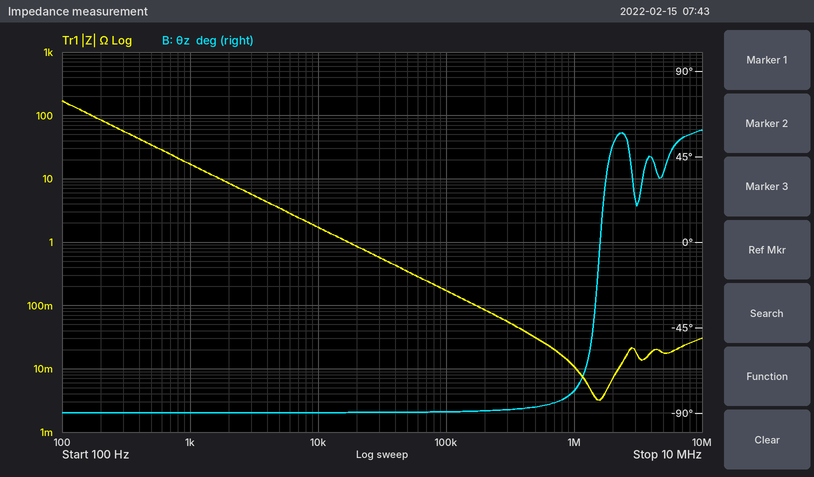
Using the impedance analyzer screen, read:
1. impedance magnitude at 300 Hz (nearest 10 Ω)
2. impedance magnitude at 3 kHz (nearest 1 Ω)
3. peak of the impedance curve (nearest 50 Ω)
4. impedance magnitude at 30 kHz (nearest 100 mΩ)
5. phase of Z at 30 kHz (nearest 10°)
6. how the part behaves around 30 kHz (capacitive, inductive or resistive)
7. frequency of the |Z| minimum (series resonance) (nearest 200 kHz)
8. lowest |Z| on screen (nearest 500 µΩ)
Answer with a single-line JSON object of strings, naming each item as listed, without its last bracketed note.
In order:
{"impedance magnitude at 300 Hz": "60 Ω", "impedance magnitude at 3 kHz": "6 Ω", "peak of the impedance curve": "150 Ω", "impedance magnitude at 30 kHz": "600 mΩ", "phase of Z at 30 kHz": "-90°", "how the part behaves around 30 kHz": "capacitive", "frequency of the |Z| minimum (series resonance)": "1.6 MHz", "lowest |Z| on screen": "3.0 mΩ"}
